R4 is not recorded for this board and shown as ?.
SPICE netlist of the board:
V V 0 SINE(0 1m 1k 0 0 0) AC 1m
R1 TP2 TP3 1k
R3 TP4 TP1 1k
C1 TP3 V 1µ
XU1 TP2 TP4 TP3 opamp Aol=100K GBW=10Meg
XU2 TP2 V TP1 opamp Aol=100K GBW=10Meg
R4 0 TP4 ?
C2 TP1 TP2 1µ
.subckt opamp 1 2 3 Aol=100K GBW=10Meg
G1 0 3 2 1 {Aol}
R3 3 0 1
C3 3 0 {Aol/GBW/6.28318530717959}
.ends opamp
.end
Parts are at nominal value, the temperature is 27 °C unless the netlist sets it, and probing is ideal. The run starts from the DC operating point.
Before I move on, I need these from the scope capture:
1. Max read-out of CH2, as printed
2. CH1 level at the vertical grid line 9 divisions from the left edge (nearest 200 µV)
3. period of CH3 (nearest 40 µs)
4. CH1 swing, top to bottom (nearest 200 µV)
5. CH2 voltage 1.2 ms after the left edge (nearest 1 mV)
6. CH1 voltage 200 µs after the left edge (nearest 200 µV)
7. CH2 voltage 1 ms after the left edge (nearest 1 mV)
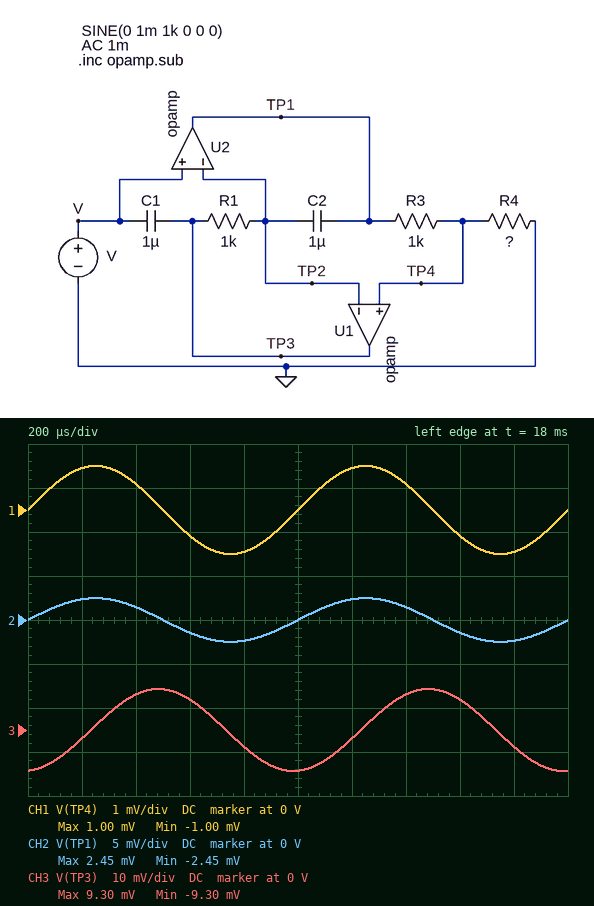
2.45 mV
-1.0 mV
1.00 ms
2.0 mV
2 mV
1.0 mV
0 V
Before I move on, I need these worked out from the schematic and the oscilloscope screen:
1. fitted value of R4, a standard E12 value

680 Ω
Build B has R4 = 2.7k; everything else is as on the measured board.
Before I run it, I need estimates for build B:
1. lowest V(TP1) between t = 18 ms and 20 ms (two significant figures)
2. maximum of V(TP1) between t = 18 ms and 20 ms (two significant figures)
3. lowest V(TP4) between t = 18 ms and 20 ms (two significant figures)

-1.4 mV
1.4 mV
-1.0 mV
